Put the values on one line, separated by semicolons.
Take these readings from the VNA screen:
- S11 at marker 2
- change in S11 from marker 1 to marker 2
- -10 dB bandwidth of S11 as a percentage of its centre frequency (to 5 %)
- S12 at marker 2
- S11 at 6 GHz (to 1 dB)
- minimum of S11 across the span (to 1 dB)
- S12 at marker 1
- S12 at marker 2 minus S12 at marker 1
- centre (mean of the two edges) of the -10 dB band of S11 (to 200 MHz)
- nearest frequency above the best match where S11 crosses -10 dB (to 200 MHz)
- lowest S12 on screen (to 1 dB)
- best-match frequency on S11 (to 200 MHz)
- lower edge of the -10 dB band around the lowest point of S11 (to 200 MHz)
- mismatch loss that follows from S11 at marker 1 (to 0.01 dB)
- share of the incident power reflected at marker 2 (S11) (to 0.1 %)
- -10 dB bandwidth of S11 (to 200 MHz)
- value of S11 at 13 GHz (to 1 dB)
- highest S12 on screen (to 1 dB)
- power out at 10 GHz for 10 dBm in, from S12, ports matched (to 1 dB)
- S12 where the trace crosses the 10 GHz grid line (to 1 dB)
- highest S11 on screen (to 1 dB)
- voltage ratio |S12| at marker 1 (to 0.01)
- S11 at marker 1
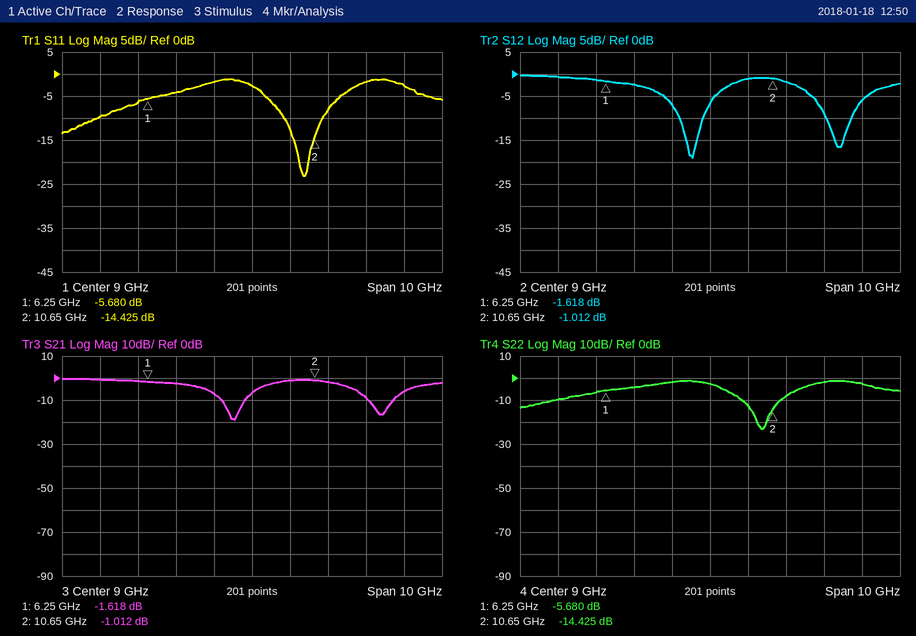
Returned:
-14.425 dB; -8.745 dB; 10 %; -1.012 dB; -6 dB; -23 dB; -1.618 dB; 0.606 dB; 10.4 GHz; 10.8 GHz; -19 dB; 10.4 GHz; 9.8 GHz; 1.37 dB; 3.6 %; 1.0 GHz; -3 dB; 0 dB; 9 dBm; -1 dB; -1 dB; 0.83; -5.680 dB
